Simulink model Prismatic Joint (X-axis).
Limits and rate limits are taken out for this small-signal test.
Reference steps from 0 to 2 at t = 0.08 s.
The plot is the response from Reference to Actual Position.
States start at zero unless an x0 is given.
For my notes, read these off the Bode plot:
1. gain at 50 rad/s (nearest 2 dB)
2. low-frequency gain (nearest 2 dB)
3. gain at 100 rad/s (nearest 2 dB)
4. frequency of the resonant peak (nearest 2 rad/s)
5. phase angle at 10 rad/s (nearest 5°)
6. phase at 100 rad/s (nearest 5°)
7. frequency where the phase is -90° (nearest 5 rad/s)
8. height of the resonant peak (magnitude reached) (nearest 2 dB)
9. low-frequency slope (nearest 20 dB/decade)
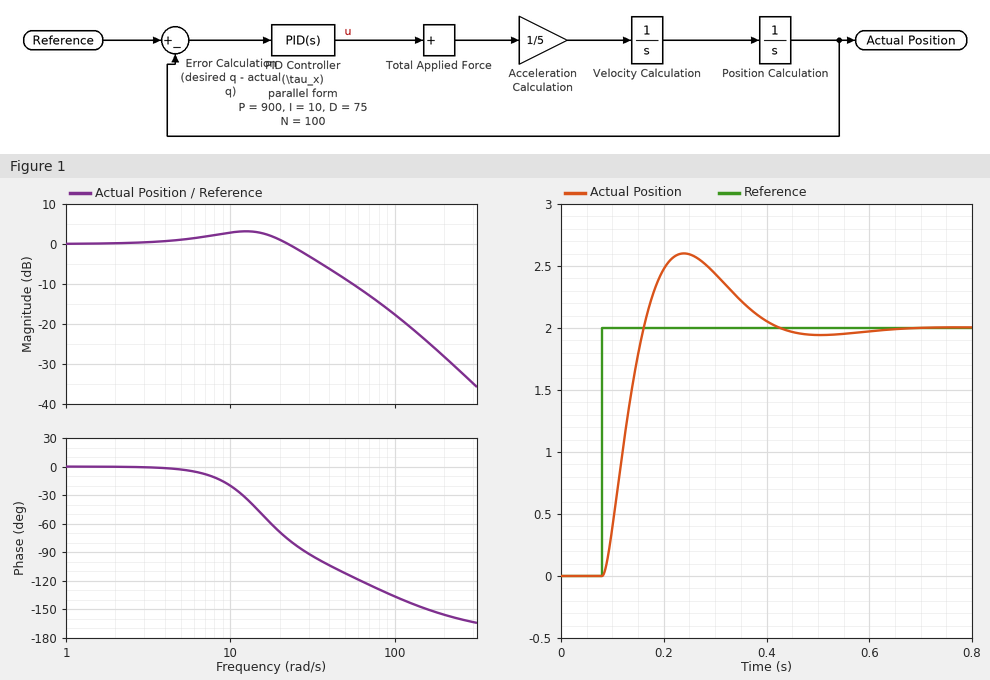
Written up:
-8 dB
0 dB
-18 dB
12 rad/s
-20°
-135°
30 rad/s
4 dB
0 dB/decade
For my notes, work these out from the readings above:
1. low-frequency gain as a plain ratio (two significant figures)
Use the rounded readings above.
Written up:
1.0
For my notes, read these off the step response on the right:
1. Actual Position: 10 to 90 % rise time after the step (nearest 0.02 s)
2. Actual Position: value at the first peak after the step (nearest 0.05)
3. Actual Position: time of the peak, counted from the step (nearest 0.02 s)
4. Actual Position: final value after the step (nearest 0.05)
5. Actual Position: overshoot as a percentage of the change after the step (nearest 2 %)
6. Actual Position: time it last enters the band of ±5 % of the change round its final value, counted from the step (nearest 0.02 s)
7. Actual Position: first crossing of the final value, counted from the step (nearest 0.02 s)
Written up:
0.06 s
2.60
0.16 s
2.00
30 %
0.30 s
0.08 s
